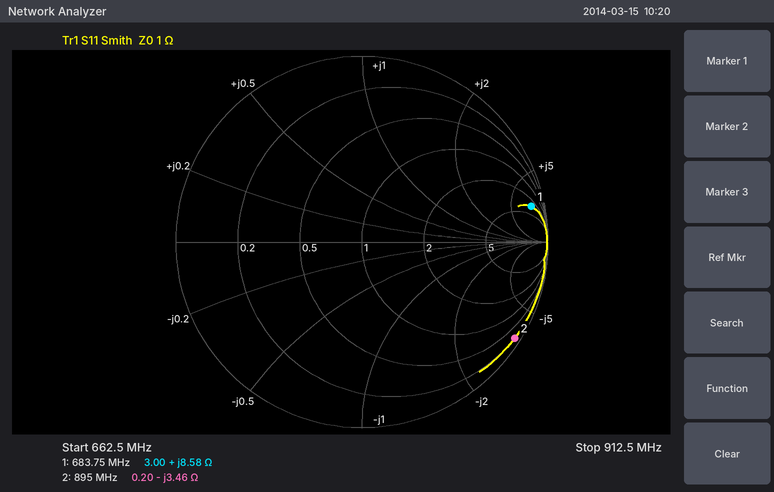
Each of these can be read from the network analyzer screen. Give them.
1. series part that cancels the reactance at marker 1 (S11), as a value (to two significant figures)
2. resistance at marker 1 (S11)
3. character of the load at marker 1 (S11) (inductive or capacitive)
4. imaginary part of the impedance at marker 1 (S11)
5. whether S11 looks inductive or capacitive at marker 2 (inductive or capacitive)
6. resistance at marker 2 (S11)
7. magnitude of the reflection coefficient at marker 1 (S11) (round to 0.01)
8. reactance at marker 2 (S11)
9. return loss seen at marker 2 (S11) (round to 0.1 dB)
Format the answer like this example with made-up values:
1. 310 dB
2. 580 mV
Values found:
1. 27 pF
2. 3.00 Ω
3. inductive
4. +8.58 Ω
5. capacitive
6. 0.20 Ω
7. 0.93
8. -3.46 Ω
9. 0.3 dB
